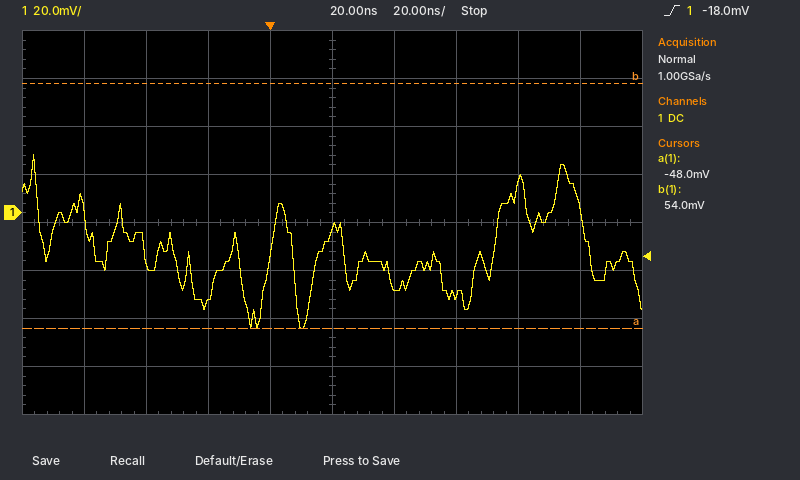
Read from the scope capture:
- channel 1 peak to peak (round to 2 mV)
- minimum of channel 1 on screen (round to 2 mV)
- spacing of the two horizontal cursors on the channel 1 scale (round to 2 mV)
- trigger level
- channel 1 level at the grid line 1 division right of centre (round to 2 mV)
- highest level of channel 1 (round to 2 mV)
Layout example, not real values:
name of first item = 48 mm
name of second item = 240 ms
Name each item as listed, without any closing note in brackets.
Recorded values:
channel 1 peak to peak = 72 mV
minimum of channel 1 on screen = -48 mV
spacing of the two horizontal cursors on the channel 1 scale = 102 mV
trigger level = -18.0 mV
channel 1 level at the grid line 1 division right of centre = -30 mV
highest level of channel 1 = 24 mV
